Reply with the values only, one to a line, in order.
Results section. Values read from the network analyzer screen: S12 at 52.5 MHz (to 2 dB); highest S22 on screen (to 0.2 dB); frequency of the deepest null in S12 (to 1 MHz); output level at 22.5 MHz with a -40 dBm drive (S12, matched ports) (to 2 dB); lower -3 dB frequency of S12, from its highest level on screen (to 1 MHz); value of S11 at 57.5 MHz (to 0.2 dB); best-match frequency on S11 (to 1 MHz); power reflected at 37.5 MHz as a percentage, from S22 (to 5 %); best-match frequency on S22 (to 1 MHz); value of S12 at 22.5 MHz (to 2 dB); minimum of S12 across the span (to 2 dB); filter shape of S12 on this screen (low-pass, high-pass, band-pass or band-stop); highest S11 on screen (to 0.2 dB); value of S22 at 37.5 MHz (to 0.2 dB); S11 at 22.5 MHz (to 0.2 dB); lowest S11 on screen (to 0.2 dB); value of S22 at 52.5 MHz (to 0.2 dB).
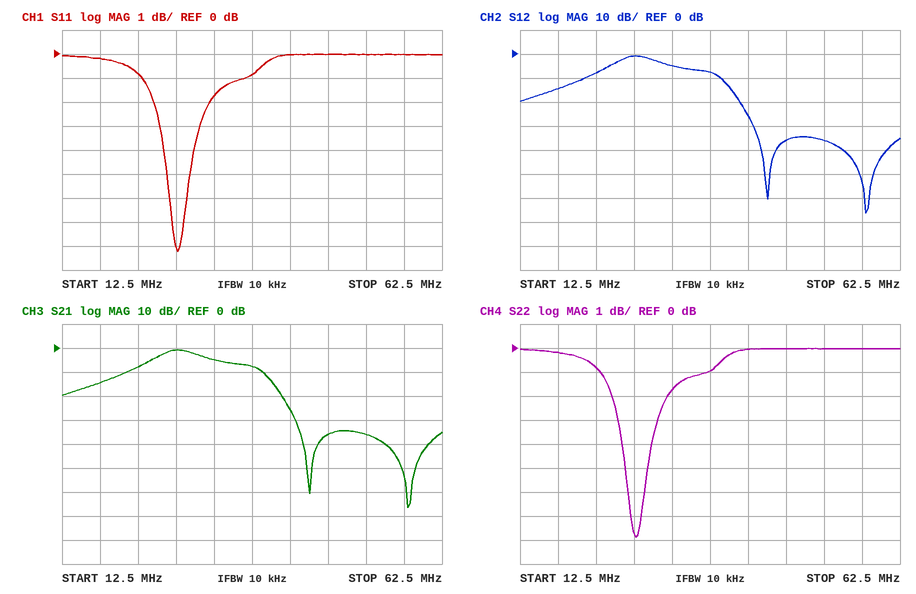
-36 dB
0.0 dB
58 MHz
-48 dBm
25 MHz
0.0 dB
28 MHz
80 %
28 MHz
-8 dB
-66 dB
band-pass
0.0 dB
-1.0 dB
-0.8 dB
-8.2 dB
0.0 dB
